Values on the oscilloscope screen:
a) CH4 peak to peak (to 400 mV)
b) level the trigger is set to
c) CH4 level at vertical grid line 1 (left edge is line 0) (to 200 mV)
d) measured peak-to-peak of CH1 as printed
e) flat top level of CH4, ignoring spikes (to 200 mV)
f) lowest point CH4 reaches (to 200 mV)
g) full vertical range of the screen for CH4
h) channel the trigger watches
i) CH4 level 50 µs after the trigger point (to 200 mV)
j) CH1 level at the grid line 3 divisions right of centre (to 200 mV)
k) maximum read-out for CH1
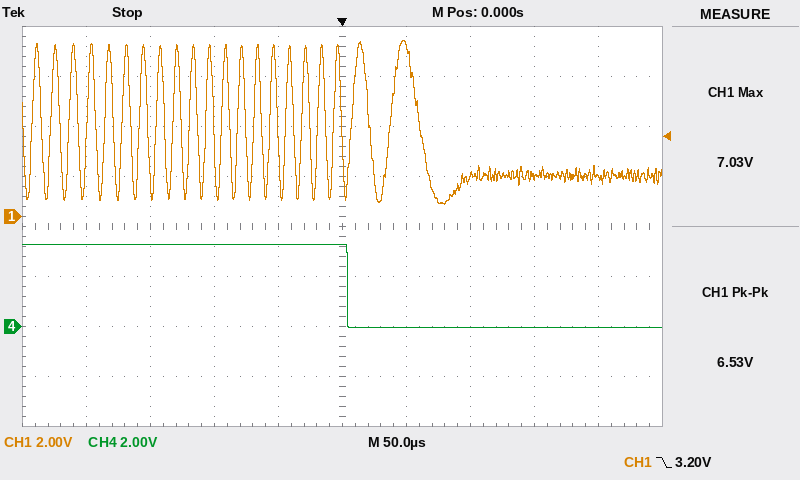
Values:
3.2 V
3.20 V
3.2 V
6.53 V
3.2 V
0.0 V
16 V
CH1
0.0 V
1.6 V
7.03 V
